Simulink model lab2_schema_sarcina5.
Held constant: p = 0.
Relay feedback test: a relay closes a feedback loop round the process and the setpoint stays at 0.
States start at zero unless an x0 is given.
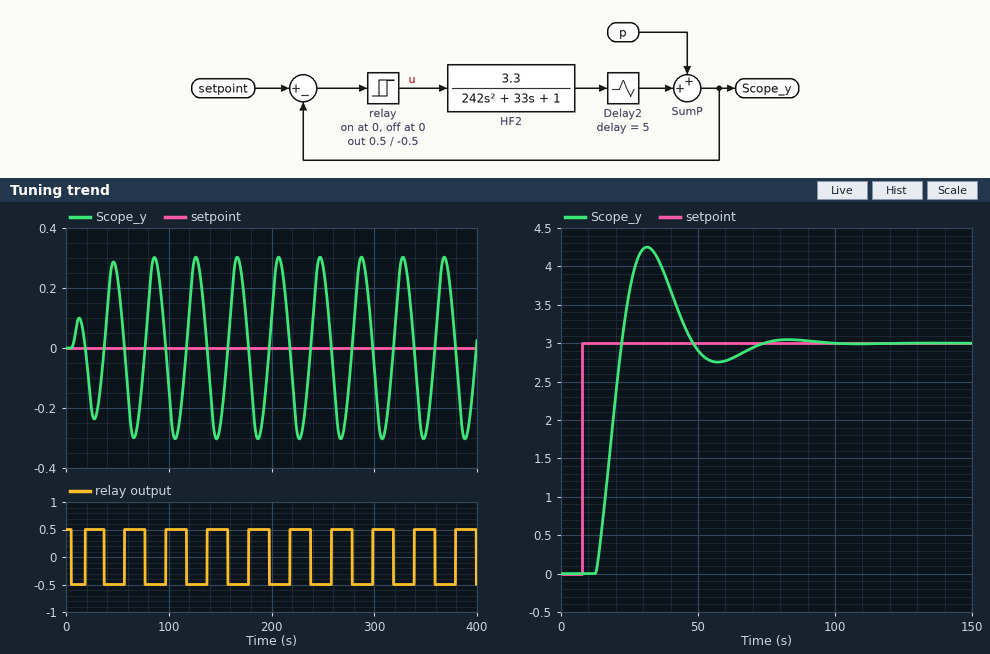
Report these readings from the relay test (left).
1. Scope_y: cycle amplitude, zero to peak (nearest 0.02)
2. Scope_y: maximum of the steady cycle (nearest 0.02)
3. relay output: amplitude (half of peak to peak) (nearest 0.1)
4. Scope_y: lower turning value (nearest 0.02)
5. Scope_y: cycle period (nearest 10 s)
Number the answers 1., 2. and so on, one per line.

1. 0.30
2. 0.30
3. 0.5
4. -0.30
5. 40 s
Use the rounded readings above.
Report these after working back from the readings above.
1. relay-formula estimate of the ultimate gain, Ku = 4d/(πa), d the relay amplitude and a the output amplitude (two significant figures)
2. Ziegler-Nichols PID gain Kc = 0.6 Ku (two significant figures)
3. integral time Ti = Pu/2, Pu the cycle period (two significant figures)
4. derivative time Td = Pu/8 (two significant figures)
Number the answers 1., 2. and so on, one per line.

1. 2.1
2. 1.3
3. 20 s
4. 5.0 s
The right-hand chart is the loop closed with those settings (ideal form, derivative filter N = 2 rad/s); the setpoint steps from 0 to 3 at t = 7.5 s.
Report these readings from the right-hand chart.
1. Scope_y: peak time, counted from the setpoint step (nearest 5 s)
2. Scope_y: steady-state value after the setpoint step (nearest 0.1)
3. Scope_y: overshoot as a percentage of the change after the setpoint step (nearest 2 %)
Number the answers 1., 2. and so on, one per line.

1. 25 s
2. 3.0
3. 42 %
